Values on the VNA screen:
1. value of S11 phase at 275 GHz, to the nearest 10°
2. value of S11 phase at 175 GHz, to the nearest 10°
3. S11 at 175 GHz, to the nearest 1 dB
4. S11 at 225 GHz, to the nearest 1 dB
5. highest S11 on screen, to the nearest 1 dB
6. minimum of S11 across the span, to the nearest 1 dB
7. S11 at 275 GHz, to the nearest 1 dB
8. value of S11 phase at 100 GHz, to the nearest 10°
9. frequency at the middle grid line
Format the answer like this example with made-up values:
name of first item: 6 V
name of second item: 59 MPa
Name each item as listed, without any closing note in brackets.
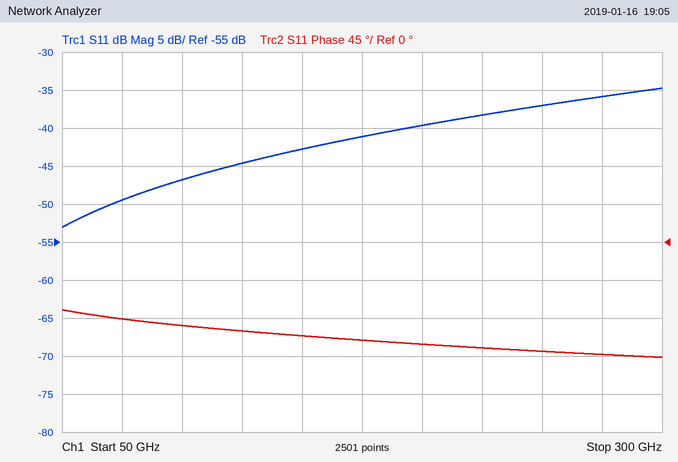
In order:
value of S11 phase at 275 GHz, to the nearest 10°: -130°
value of S11 phase at 175 GHz, to the nearest 10°: -120°
S11 at 175 GHz, to the nearest 1 dB: -41 dB
S11 at 225 GHz, to the nearest 1 dB: -38 dB
highest S11 on screen, to the nearest 1 dB: -35 dB
minimum of S11 across the span, to the nearest 1 dB: -53 dB
S11 at 275 GHz, to the nearest 1 dB: -36 dB
value of S11 phase at 100 GHz, to the nearest 10°: -100°
frequency at the middle grid line: 175 GHz
